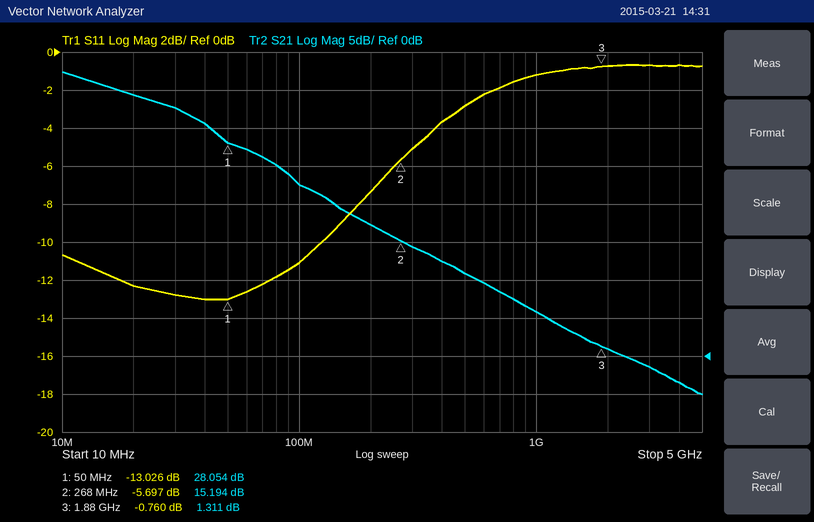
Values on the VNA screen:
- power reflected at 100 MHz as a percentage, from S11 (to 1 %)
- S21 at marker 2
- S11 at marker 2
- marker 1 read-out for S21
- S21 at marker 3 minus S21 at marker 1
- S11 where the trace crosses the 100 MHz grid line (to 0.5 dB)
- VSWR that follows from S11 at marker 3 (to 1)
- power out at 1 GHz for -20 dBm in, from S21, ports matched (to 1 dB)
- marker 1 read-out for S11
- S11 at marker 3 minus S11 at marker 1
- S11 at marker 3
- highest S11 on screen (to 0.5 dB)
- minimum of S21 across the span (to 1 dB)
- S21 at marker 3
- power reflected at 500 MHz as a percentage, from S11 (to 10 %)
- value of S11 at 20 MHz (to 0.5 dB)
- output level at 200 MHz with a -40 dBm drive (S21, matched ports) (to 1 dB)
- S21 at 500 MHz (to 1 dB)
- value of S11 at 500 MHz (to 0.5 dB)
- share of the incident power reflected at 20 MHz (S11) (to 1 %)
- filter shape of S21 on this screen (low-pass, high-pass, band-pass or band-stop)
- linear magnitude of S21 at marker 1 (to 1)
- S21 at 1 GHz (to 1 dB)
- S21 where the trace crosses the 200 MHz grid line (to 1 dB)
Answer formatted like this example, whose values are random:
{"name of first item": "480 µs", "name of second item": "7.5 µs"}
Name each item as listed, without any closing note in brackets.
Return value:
{"power reflected at 100 MHz as a percentage, from S11": "8 %", "S21 at marker 2": "15.194 dB", "S11 at marker 2": "-5.697 dB", "marker 1 read-out for S21": "28.054 dB", "S21 at marker 3 minus S21 at marker 1": "-26.743 dB", "S11 where the trace crosses the 100 MHz grid line": "-11.0 dB", "VSWR that follows from S11 at marker 3": "23", "power out at 1 GHz for -20 dBm in, from S21, ports matched": "-14 dBm", "marker 1 read-out for S11": "-13.026 dB", "S11 at marker 3 minus S11 at marker 1": "12.266 dB", "S11 at marker 3": "-0.760 dB", "highest S11 on screen": "-0.5 dB", "minimum of S21 across the span": "-5 dB", "S21 at marker 3": "1.311 dB", "power reflected at 500 MHz as a percentage, from S11": "50 %", "value of S11 at 20 MHz": "-12.5 dB", "output level at 200 MHz with a -40 dBm drive (S21, matched ports)": "-23 dBm", "S21 at 500 MHz": "11 dB", "value of S11 at 500 MHz": "-3.0 dB", "share of the incident power reflected at 20 MHz (S11)": "6 %", "filter shape of S21 on this screen": "low-pass", "linear magnitude of S21 at marker 1": "25", "S21 at 1 GHz": "6 dB", "S21 where the trace crosses the 200 MHz grid line": "17 dB"}
